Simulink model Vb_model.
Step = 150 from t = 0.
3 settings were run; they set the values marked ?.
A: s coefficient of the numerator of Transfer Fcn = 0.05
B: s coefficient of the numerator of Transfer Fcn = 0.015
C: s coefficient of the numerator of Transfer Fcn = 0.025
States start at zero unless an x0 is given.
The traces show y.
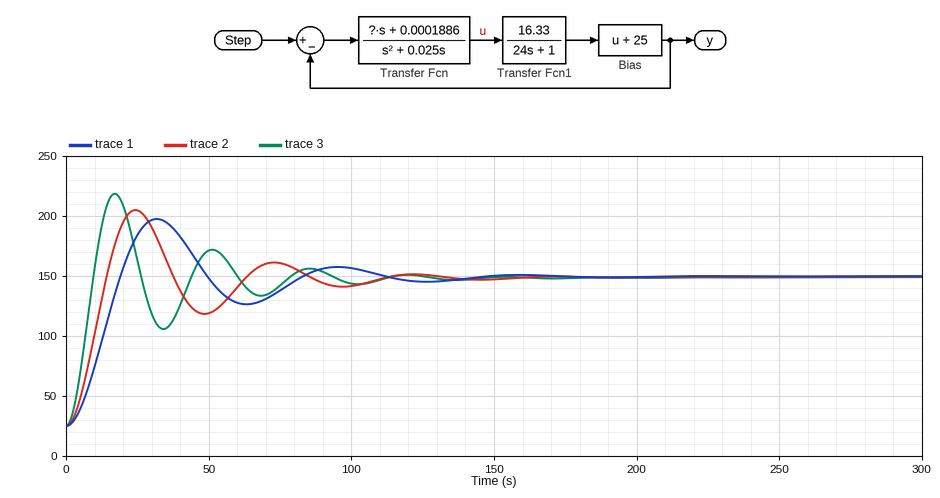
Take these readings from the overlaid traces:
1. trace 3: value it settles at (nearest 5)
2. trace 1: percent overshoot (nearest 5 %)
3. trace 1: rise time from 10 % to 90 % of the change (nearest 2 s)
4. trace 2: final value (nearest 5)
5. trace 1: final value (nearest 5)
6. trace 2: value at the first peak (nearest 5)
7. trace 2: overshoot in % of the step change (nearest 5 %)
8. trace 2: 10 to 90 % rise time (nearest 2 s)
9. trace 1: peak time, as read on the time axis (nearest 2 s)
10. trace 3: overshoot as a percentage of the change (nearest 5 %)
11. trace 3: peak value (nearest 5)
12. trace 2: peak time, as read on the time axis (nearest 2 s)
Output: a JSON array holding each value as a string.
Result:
["150", "40 %", "12 s", "150", "150", "205", "45 %", "10 s", "32 s", "55 %", "220", "24 s"]
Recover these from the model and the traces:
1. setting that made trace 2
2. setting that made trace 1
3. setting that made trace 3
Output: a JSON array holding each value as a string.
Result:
["C", "B", "A"]
